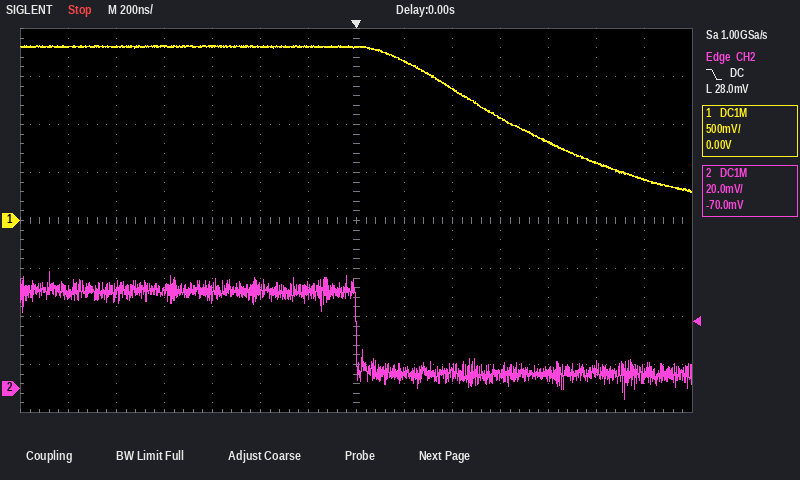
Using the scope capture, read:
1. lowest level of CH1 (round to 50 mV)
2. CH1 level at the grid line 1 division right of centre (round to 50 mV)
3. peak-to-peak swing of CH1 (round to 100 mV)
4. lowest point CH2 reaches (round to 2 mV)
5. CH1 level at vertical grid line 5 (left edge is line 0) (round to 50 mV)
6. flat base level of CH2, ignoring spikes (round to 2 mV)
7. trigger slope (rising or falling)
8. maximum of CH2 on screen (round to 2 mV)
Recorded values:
300 mV
1.65 V
1.50 V
-4 mV
1.80 V
6 mV
falling
48 mV
